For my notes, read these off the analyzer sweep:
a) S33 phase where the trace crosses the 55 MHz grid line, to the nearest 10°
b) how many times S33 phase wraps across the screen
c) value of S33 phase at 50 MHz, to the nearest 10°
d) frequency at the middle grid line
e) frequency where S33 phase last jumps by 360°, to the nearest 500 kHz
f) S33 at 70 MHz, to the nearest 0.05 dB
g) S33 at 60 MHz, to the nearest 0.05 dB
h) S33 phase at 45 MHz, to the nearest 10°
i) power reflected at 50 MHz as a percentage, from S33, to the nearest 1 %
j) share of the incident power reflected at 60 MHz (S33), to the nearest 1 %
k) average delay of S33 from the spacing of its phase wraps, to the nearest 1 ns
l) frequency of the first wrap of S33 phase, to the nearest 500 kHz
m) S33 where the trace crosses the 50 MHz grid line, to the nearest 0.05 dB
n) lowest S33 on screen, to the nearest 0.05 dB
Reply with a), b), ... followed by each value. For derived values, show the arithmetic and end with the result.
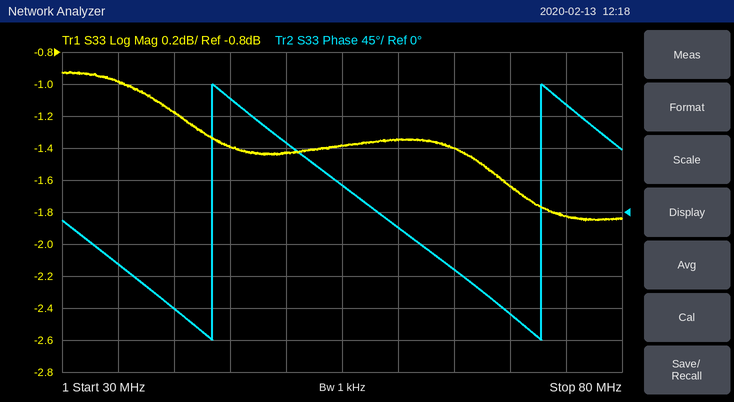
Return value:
a) 40°
b) 2
c) 100°
d) 55 MHz
e) 73.0 MHz
f) -1.65 dB
g) -1.35 dB
h) 160°
i) 10^(-1.45/10) ≈ 72 %
j) 10^(-1.35/10) ≈ 73 %
k) 1 cycle / (73.0 MHz − 43.5 MHz) ≈ 34 ns
l) 43.5 MHz
m) -1.45 dB
n) -1.85 dB
